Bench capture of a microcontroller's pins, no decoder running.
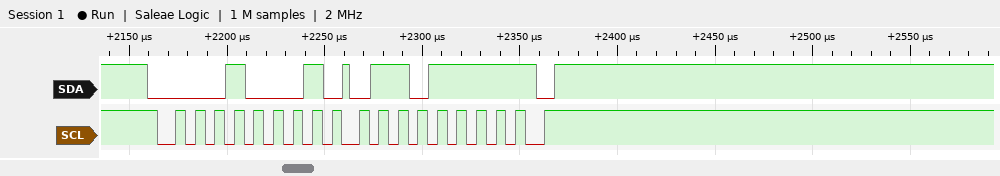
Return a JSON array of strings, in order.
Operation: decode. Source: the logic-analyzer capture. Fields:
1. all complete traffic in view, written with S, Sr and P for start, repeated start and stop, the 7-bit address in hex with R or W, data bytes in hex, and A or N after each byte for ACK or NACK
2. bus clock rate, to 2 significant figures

["S 08R A 6F N P", "100 kHz"]
